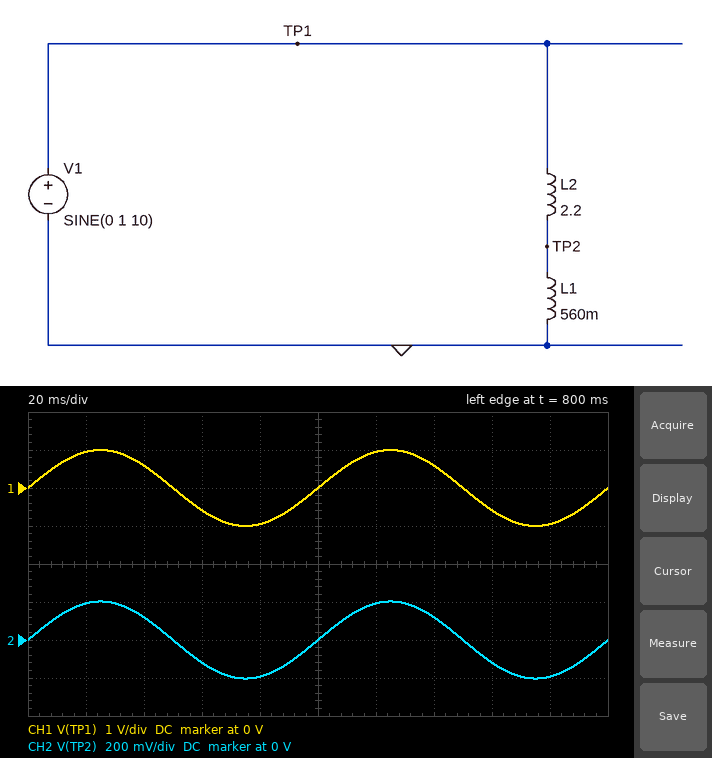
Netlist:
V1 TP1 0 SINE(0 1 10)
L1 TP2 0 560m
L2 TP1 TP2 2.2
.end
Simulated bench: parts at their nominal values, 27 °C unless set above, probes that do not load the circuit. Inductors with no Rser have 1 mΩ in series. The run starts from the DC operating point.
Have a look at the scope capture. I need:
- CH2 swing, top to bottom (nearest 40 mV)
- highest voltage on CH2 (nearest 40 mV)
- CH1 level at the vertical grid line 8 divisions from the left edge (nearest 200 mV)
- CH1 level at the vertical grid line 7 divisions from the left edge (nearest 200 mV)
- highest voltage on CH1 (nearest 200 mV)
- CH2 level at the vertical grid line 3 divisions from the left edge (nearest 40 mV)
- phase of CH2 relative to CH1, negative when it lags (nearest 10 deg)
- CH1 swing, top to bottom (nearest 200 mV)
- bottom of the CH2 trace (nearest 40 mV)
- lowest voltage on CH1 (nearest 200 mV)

400 mV
200 mV
-600 mV
600 mV
1.0 V
-120 mV
0 deg
2.0 V
-200 mV
-1.0 V
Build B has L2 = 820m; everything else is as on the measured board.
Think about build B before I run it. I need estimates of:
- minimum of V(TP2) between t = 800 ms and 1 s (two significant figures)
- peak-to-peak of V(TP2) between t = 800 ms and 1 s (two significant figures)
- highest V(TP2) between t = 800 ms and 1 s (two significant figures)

-410 mV
810 mV
410 mV
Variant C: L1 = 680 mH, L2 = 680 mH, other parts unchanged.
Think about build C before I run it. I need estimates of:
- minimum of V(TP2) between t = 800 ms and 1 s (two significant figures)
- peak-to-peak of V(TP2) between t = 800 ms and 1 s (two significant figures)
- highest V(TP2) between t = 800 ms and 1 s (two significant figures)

-500 mV
1.0 V
500 mV
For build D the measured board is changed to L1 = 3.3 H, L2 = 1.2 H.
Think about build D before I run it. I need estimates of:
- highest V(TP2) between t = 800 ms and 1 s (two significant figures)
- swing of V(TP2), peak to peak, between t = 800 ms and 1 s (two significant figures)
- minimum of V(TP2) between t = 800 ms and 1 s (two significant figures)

730 mV
1.5 V
-730 mV
